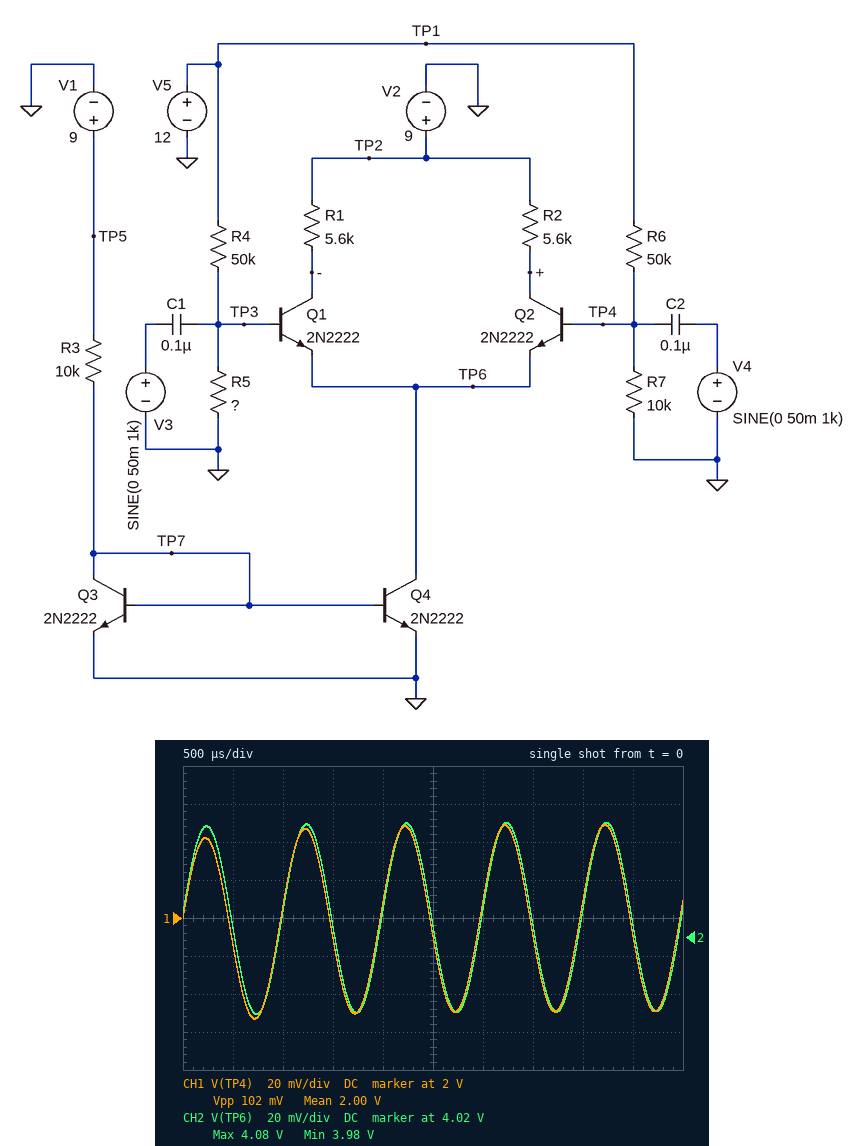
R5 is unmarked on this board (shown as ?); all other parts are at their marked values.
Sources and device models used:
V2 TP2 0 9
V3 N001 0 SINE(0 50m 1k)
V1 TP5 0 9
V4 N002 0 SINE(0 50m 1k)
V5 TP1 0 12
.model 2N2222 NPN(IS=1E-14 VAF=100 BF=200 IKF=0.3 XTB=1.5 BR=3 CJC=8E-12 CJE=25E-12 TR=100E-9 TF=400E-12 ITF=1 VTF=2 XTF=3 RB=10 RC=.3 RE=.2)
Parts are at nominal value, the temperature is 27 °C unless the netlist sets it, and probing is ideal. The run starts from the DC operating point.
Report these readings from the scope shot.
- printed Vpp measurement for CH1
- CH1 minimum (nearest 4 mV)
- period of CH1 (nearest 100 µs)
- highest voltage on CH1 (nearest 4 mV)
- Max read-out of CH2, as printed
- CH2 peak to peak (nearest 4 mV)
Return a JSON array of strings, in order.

["102 mV", "1.948 V", "1.0 ms", "2.048 V", "4.08 V", "100 mV"]
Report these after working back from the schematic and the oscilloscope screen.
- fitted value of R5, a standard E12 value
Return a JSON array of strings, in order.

["33 kΩ"]
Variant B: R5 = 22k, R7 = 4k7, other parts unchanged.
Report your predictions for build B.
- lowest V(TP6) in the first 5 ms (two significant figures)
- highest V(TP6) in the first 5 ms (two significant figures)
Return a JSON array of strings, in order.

["2.9 V", "3.0 V"]
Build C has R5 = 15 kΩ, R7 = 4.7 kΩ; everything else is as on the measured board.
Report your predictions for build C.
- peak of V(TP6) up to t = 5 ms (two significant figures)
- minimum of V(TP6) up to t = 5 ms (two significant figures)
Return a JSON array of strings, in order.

["2.1 V", "2.0 V"]
